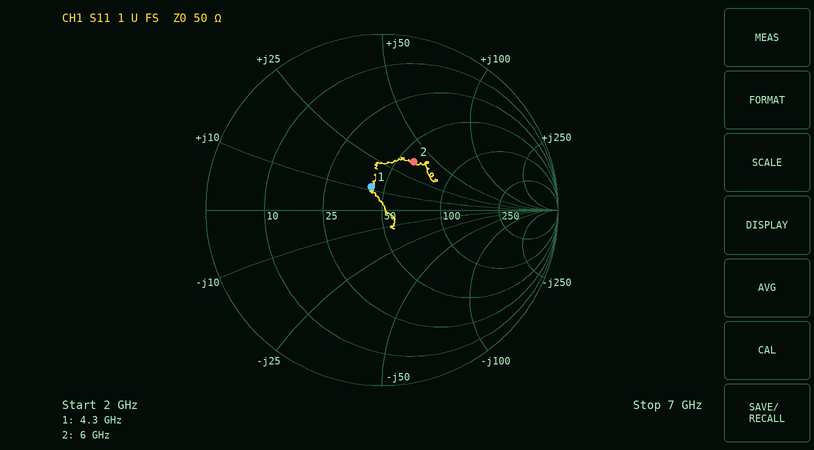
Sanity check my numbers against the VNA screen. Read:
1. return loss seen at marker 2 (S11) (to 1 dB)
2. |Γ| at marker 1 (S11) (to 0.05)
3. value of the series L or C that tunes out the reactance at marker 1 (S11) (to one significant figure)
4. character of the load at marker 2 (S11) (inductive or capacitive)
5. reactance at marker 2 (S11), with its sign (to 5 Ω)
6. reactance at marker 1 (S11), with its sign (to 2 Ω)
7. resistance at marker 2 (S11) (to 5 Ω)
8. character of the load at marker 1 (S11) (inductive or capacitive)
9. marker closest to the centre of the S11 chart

10 dB
0.15
3 pF
inductive
+35 Ω
+12 Ω
60 Ω
inductive
marker 1
